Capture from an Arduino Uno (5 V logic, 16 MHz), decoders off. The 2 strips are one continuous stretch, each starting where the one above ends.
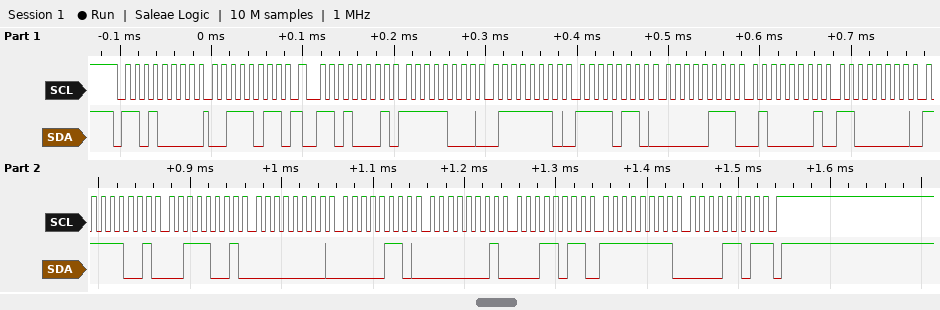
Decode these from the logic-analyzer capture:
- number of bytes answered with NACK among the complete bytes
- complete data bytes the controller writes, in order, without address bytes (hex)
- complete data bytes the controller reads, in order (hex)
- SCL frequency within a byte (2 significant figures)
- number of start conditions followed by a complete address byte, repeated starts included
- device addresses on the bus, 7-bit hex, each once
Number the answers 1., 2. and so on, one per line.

1. 1
2. 3B
3. F8 7E F6 07 41 C0 F9 39 00 06 01 1B FF 0D
4. 100 kHz
5. 2
6. 0x68
